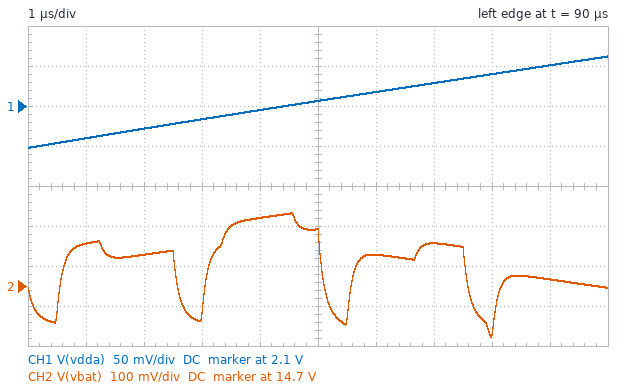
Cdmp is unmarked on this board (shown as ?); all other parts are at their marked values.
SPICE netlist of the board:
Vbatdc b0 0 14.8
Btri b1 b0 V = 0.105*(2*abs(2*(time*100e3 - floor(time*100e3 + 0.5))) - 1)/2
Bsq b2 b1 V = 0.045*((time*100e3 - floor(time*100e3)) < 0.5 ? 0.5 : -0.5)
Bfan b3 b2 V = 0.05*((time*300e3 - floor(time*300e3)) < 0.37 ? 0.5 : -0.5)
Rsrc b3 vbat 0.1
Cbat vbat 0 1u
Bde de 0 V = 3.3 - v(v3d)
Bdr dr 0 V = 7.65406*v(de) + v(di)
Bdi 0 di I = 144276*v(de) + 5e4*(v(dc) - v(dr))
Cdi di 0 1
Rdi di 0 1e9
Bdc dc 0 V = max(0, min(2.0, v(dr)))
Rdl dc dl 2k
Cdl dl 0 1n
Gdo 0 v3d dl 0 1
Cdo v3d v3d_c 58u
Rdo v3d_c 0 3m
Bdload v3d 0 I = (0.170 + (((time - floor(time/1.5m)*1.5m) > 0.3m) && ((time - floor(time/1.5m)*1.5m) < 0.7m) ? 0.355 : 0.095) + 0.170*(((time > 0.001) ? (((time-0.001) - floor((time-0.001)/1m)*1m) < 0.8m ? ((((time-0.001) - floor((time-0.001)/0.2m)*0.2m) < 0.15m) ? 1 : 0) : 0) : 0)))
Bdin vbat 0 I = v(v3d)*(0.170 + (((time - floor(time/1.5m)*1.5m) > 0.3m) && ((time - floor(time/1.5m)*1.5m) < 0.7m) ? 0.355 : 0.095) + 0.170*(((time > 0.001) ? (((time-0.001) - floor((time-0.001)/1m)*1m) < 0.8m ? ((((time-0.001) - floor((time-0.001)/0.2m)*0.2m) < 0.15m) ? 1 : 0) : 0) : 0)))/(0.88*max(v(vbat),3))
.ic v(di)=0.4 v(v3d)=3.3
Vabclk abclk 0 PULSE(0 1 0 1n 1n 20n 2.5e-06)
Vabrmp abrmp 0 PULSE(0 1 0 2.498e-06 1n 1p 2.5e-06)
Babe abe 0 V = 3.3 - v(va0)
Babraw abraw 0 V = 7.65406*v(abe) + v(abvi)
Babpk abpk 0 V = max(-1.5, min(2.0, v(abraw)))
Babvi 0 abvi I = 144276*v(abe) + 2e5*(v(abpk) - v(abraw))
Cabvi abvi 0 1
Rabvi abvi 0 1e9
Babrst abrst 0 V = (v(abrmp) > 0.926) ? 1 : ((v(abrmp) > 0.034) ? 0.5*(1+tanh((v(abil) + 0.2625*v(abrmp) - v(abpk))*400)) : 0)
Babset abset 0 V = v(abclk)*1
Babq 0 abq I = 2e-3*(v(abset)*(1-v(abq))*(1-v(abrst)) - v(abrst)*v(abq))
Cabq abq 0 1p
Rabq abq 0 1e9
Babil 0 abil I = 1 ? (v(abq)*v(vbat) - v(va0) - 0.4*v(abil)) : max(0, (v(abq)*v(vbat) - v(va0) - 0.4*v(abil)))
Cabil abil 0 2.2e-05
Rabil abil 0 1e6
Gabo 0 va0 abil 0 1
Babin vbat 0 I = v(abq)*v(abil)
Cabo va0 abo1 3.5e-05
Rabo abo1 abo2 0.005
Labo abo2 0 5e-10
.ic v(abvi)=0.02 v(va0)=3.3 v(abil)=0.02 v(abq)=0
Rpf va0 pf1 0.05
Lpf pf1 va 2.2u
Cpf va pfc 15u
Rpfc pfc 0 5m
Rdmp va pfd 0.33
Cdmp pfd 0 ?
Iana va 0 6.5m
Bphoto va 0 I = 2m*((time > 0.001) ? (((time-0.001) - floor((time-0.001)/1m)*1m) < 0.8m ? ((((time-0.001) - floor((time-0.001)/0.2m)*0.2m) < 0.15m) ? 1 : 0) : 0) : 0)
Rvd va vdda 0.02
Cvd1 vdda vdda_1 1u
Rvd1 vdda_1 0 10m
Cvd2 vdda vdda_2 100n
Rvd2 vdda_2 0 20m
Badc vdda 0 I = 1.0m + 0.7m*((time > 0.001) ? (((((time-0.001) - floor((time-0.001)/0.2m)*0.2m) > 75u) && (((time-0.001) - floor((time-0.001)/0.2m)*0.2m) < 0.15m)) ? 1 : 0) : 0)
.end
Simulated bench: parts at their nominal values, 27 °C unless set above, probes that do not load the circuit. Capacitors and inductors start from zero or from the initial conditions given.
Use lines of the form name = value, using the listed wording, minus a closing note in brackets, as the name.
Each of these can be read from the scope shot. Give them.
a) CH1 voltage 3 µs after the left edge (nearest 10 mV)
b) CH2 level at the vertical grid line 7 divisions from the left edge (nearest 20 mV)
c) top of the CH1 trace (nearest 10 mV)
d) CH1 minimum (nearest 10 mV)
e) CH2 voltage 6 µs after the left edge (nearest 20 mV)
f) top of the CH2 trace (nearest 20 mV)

CH1 voltage 3 µs after the left edge = 2.08 V
CH2 level at the vertical grid line 7 divisions from the left edge = 14.80 V
top of the CH1 trace = 2.16 V
CH1 minimum = 2.05 V
CH2 voltage 6 µs after the left edge = 14.78 V
top of the CH2 trace = 14.88 V
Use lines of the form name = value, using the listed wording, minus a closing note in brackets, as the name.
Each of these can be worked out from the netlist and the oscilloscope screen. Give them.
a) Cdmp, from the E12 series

Cdmp, from the E12 series = 100 µF
